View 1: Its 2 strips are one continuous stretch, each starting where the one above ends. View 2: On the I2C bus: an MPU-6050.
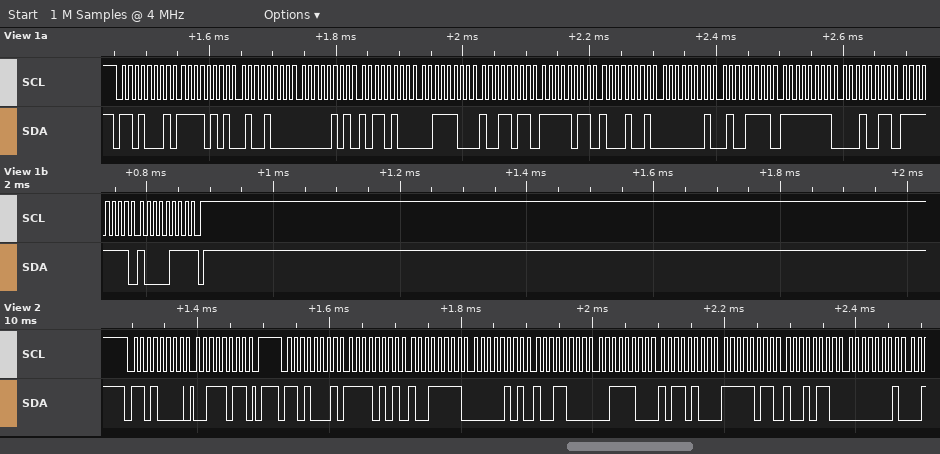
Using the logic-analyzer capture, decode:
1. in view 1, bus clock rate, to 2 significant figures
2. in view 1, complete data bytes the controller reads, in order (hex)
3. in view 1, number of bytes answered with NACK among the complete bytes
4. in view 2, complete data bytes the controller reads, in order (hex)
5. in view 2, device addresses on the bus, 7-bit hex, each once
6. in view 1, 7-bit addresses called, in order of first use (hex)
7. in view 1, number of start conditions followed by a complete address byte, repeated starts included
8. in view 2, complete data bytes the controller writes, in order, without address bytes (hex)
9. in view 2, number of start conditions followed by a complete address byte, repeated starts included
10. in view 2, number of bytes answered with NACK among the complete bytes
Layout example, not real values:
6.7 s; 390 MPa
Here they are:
100 kHz; F5 48 05 B4 3C 9B FB 89 01 4F FF 13 FF 87; 1; F5 9F 05 98 3C B4 FB 96 01; 0x68; 0x68; 1; 3B; 2; 0
